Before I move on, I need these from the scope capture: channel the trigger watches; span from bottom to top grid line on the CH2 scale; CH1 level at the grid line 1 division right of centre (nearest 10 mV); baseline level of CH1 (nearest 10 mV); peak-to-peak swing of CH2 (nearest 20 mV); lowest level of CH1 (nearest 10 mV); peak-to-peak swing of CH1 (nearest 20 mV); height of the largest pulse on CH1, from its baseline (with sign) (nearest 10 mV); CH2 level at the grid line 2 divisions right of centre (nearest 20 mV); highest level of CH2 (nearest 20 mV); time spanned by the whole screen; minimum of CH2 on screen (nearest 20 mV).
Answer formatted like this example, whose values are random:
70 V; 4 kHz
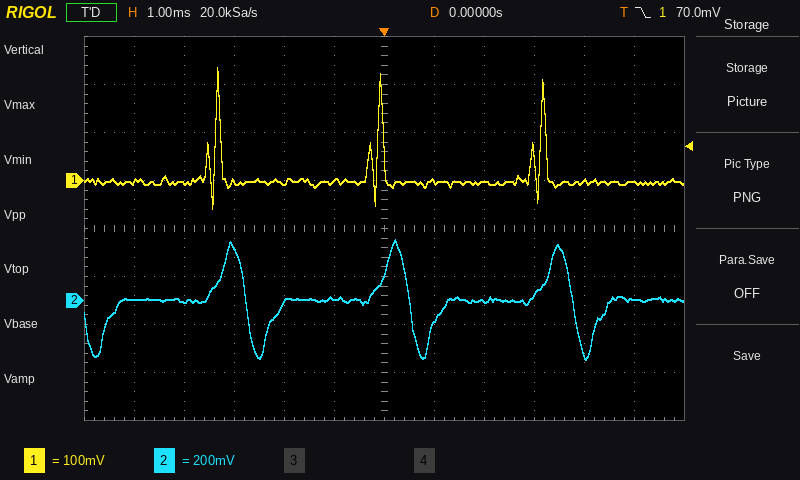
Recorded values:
CH1; 1.6 V; 0 mV; 0 mV; 500 mV; -60 mV; 300 mV; +240 mV; 0 mV; 260 mV; 12 ms; -240 mV
